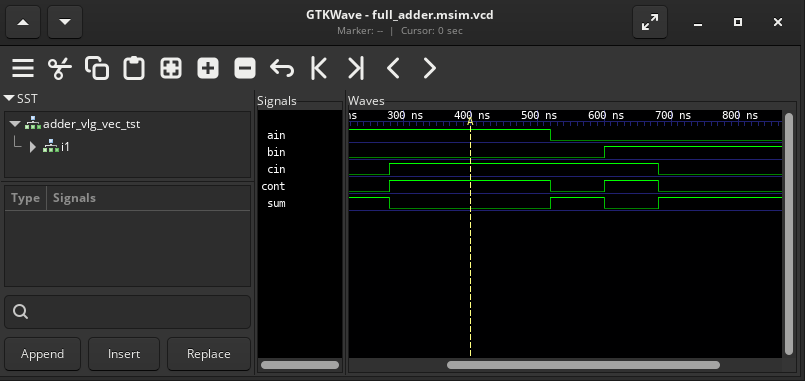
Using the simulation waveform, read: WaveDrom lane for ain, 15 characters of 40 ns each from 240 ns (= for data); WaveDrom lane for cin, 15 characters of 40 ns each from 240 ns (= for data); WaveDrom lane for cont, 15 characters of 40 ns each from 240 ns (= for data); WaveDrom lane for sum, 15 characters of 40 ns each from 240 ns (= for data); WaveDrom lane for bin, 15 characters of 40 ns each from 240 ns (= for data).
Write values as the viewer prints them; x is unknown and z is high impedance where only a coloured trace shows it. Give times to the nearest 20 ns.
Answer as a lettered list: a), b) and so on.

a) {name: 'ain', wave: '1......0.......'}
b) {name: 'cin', wave: '01.........0...'}
c) {name: 'cont', wave: '01.....0.1.0...'}
d) {name: 'sum', wave: '10.....1.0.1...'}
e) {name: 'bin', wave: '0........1.....'}
